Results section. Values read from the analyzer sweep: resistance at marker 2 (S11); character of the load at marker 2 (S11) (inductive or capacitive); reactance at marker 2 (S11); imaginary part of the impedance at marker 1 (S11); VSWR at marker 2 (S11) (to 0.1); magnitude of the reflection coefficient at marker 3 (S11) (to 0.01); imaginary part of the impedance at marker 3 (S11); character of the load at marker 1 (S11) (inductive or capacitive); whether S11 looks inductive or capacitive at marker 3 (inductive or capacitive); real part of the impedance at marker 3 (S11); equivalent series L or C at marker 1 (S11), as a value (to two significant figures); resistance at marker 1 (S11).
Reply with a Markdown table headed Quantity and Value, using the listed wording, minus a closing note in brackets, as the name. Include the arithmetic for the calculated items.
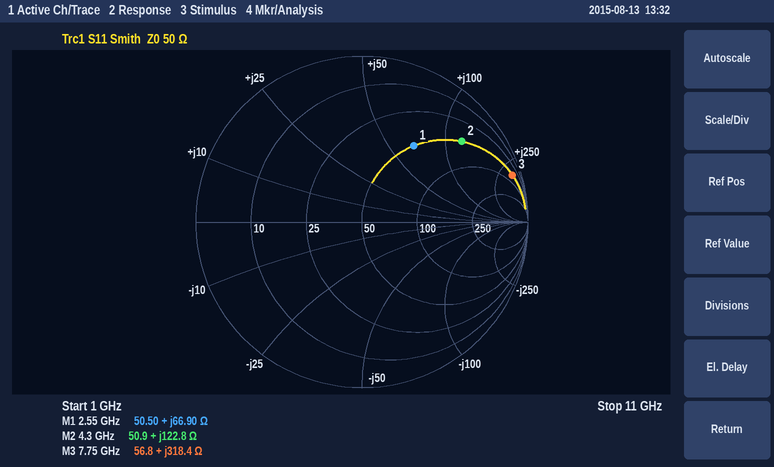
| Quantity | Value |
|---|---|
| resistance at marker 2 | 50.9 Ω |
| character of the load at marker 2 (S11) | inductive |
| reactance at marker 2 | +122.8 Ω |
| imaginary part of the impedance at marker 1 | +66.90 Ω |
| VSWR at marker 2 (S11) | 7.8 |
| magnitude of the reflection coefficient at marker 3 (S11) | 0.95 |
| imaginary part of the impedance at marker 3 | +318.4 Ω |
| character of the load at marker 1 (S11) | inductive |
| whether S11 looks inductive or capacitive at marker 3 | inductive |
| real part of the impedance at marker 3 | 56.8 Ω |
| equivalent series L or C at marker 1 (S11), as a value | L = 66.9 Ω/(2π × 2.55 GHz) ≈ 4.2 nH |
| resistance at marker 1 | 50.50 Ω |
